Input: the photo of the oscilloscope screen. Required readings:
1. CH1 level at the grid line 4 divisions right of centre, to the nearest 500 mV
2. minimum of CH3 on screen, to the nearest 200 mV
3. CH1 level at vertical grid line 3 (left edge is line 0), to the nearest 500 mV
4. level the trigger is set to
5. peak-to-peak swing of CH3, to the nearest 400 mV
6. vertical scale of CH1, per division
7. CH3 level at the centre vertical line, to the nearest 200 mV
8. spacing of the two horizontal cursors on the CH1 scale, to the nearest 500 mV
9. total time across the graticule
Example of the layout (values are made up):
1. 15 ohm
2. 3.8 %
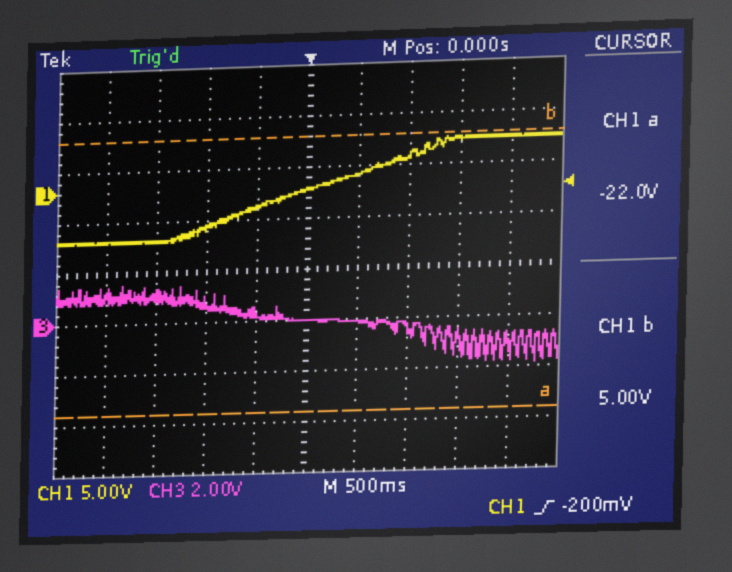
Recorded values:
1. 4.5 V
2. -1.8 V
3. -3.5 V
4. -200 mV
5. 3.2 V
6. 5 V
7. 0.0 V
8. 27.0 V
9. 5 s
